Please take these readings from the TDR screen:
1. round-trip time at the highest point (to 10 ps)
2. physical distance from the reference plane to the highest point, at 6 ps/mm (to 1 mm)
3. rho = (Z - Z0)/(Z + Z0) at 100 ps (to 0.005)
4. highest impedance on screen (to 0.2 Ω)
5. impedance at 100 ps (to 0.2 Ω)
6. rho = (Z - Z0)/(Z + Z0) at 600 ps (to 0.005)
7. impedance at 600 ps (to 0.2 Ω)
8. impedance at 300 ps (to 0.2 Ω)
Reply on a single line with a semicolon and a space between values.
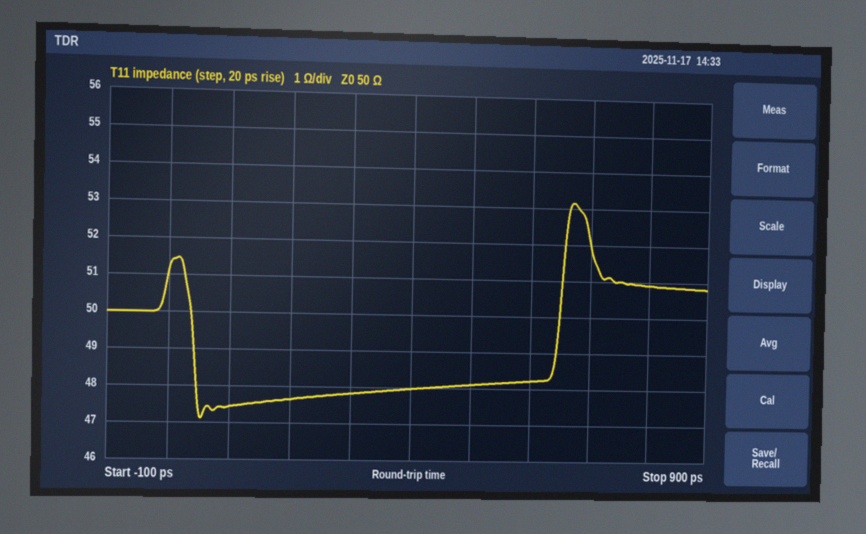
670 ps; 56 mm; -0.025; 53.2 Ω; 47.4 Ω; -0.020; 48.2 Ω; 47.8 Ω
